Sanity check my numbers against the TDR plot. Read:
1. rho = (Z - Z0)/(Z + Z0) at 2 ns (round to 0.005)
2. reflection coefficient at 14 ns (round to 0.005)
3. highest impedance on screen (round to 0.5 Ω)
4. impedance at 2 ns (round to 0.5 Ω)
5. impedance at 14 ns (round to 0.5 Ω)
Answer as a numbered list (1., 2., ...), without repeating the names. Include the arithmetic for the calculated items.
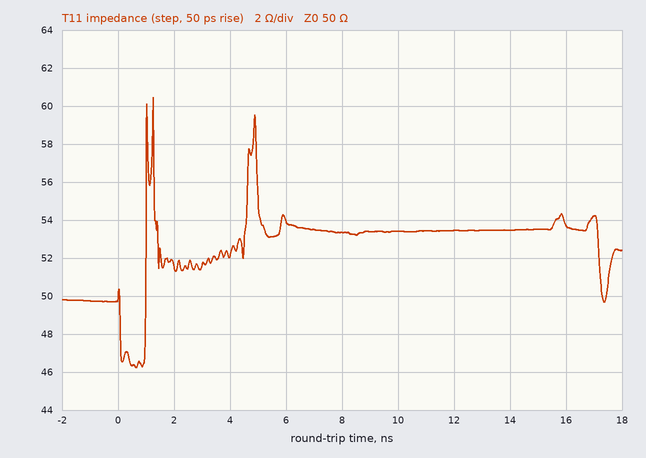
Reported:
1. (51.5 − 50)/(51.5 + 50) ≈ +0.015
2. (53.5 − 50)/(53.5 + 50) ≈ +0.0338, so +0.035 to the nearest 0.005
3. 60.5 Ω
4. 51.5 Ω
5. 53.5 Ω
